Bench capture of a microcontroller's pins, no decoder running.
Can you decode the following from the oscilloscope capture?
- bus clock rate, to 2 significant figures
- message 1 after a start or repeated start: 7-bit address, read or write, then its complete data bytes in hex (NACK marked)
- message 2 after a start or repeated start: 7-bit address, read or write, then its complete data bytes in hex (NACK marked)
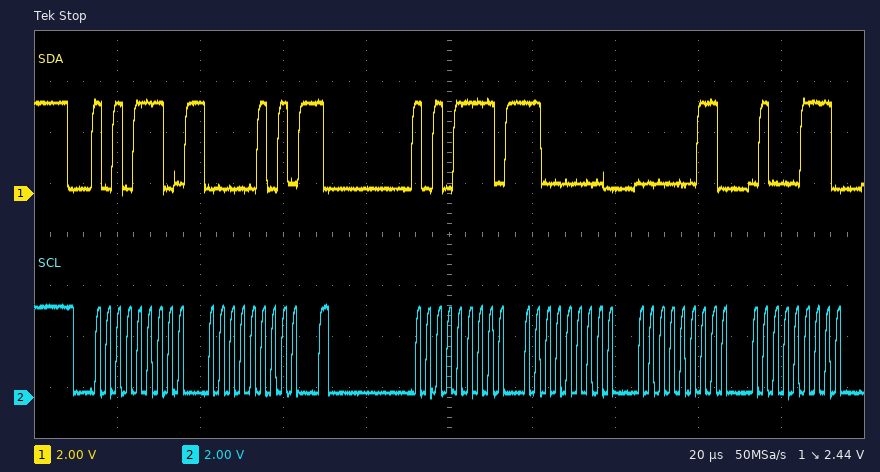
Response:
400 kHz
0x57 write: 05
0x57 read: C0 03 47
